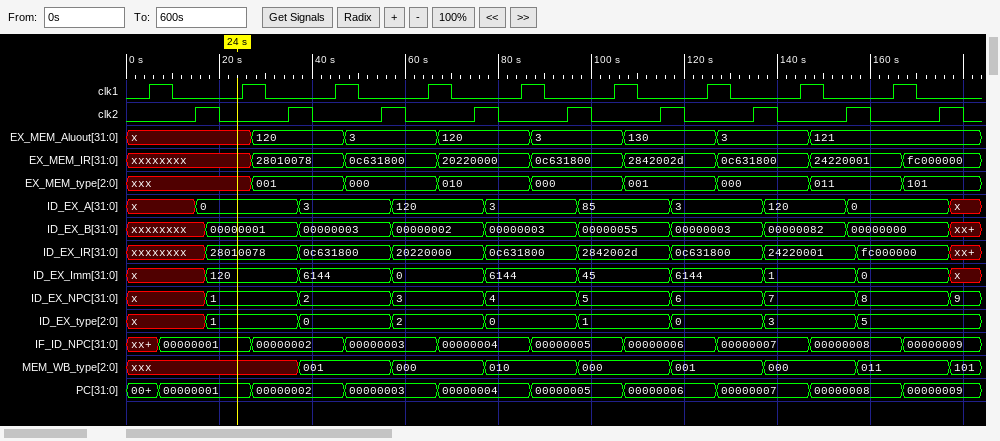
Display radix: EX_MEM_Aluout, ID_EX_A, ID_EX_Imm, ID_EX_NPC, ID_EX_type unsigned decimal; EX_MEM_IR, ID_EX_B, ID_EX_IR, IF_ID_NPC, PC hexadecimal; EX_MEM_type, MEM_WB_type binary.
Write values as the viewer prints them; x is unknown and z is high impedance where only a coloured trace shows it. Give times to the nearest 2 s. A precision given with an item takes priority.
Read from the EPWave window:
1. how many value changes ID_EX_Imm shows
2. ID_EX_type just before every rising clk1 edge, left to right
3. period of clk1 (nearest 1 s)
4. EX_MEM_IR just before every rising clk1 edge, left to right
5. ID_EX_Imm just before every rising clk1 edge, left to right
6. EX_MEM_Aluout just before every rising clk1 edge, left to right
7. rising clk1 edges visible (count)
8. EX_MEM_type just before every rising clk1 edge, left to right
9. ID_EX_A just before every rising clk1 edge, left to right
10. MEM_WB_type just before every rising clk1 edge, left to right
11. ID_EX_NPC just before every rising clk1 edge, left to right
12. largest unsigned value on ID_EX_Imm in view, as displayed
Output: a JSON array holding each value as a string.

["9", "x, 1, 0, 2, 0, 1, 0, 3, 5", "20 s", "xxxxxxxx, xxxxxxxx, 28010078, 0c631800, 20220000, 0c631800, 2842002d, 0c631800, 24220001", "x, 120, 6144, 0, 6144, 45, 6144, 1, 0", "x, x, 120, 3, 120, 3, 130, 3, 121", "9", "xxx, xxx, 001, 000, 010, 000, 001, 000, 011", "x, 0, 3, 120, 3, 85, 3, 120, 0", "xxx, xxx, 001, 000, 010, 000, 001, 000, 011", "x, 1, 2, 3, 4, 5, 6, 7, 8", "6144"]
